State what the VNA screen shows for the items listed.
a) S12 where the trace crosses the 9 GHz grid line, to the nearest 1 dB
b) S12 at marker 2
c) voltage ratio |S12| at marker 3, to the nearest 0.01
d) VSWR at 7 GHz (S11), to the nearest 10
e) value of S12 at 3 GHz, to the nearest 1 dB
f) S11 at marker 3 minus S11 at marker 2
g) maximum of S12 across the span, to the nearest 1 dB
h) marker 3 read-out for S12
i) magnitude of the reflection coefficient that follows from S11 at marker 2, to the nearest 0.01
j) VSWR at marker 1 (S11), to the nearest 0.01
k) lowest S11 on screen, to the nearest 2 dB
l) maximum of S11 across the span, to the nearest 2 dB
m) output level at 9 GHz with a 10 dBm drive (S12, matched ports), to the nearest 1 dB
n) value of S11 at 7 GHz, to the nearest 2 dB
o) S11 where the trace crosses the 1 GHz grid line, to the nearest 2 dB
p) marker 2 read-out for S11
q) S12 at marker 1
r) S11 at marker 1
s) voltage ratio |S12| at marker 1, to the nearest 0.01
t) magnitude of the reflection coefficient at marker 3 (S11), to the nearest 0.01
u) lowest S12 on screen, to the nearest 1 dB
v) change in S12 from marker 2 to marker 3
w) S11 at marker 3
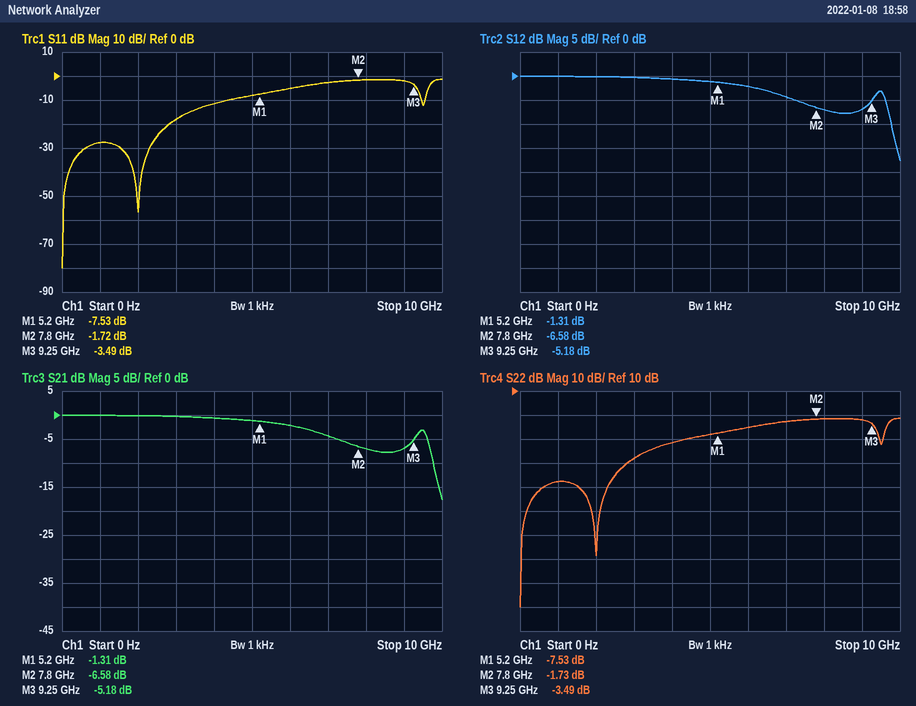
-7 dB
-6.58 dB
0.55
10
0 dB
-1.77 dB
0 dB
-5.18 dB
0.82
2.45
-80 dB
-2 dB
3 dBm
-2 dB
-28 dB
-1.72 dB
-1.31 dB
-7.53 dB
0.86
0.67
-18 dB
1.40 dB
-3.49 dB
